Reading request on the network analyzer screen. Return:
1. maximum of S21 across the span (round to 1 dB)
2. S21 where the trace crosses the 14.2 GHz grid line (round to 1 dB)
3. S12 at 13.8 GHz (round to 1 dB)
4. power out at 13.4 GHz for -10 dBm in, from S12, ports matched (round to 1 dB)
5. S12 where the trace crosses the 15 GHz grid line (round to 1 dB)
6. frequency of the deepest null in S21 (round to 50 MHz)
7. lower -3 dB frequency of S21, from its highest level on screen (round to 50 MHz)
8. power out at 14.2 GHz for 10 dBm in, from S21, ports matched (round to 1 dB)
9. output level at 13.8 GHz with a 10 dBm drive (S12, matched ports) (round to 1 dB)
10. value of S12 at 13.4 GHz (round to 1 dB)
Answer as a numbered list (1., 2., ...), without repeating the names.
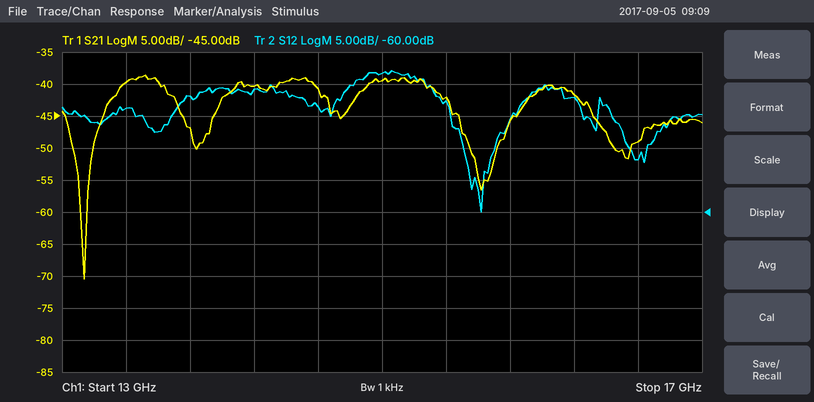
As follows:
1. -39 dB
2. -40 dB
3. -42 dB
4. -54 dBm
5. -38 dB
6. 13.15 GHz
7. 13.35 GHz
8. -30 dBm
9. -32 dBm
10. -44 dB
